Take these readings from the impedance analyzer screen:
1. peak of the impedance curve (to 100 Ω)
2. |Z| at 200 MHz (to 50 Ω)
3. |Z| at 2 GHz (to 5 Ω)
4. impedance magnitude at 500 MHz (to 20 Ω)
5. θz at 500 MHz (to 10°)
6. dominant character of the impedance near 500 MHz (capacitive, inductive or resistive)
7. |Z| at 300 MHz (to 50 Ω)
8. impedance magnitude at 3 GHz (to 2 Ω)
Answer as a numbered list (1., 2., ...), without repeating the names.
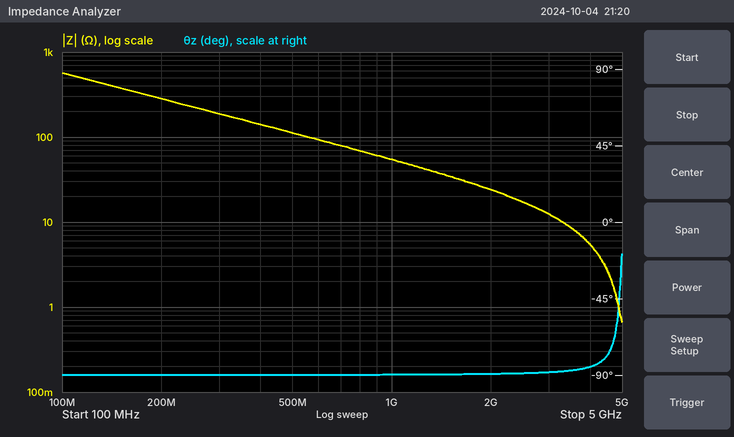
1. 600 Ω
2. 300 Ω
3. 25 Ω
4. 120 Ω
5. -90°
6. capacitive
7. 200 Ω
8. 12 Ω
